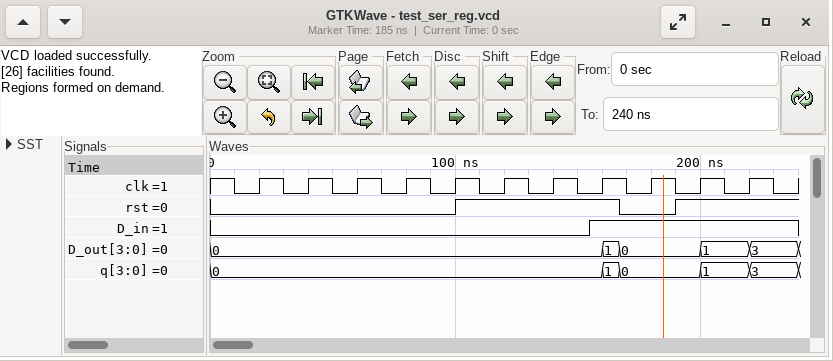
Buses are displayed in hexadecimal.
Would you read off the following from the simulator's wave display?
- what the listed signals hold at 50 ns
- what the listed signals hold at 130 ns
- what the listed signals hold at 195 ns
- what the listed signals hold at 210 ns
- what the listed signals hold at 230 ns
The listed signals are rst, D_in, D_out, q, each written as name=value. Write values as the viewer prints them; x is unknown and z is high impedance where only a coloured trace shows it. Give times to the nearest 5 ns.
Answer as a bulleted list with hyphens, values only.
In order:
- rst=0, D_in=0, D_out=0, q=0
- rst=1, D_in=0, D_out=0, q=0
- rst=1, D_in=1, D_out=0, q=0
- rst=1, D_in=1, D_out=1, q=1
- rst=1, D_in=1, D_out=3, q=3
